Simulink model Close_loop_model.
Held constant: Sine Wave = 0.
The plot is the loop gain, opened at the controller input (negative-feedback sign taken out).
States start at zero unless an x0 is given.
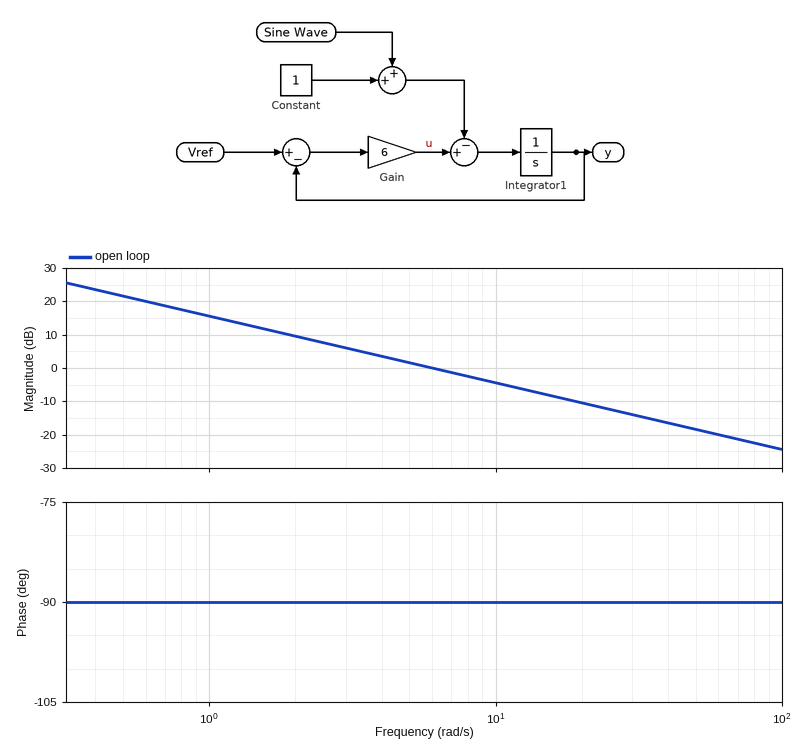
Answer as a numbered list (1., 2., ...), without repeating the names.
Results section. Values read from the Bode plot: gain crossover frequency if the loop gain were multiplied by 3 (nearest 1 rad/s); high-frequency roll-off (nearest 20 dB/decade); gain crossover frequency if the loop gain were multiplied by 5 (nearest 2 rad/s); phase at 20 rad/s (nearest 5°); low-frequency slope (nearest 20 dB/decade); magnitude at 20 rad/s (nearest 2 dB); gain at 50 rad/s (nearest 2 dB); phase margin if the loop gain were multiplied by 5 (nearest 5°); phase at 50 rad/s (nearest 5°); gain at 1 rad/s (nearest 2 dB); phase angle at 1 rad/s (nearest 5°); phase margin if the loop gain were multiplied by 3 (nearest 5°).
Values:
1. 18 rad/s
2. -20 dB/decade
3. 30 rad/s
4. -90°
5. -20 dB/decade
6. -10 dB
7. -18 dB
8. 90°
9. -90°
10. 16 dB
11. -90°
12. 90°
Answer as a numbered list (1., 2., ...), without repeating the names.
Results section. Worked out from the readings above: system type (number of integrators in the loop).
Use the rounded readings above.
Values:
1. 1
